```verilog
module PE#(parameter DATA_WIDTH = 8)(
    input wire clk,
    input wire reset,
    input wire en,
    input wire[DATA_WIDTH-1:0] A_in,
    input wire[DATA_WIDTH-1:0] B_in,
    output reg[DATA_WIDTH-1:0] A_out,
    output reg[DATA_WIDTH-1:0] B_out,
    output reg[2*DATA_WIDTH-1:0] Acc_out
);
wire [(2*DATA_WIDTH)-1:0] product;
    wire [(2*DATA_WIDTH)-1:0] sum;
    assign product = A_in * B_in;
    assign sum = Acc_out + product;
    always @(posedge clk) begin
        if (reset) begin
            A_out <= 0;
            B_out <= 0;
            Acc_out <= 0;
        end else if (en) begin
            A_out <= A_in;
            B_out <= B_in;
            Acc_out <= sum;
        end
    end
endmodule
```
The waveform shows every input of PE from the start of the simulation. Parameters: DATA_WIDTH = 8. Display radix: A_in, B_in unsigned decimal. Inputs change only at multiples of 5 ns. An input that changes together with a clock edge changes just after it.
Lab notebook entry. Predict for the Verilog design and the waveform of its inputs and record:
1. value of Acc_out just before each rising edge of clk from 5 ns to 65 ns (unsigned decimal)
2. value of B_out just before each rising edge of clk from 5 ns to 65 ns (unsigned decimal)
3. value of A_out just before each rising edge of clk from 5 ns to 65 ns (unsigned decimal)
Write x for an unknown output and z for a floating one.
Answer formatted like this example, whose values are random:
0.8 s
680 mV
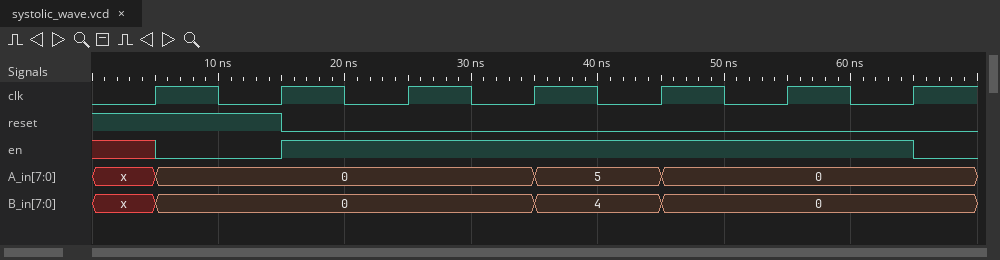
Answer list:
x, 0, 0, 0, 0, 20, 20
x, 0, 0, 0, 0, 4, 0
x, 0, 0, 0, 0, 5, 0
